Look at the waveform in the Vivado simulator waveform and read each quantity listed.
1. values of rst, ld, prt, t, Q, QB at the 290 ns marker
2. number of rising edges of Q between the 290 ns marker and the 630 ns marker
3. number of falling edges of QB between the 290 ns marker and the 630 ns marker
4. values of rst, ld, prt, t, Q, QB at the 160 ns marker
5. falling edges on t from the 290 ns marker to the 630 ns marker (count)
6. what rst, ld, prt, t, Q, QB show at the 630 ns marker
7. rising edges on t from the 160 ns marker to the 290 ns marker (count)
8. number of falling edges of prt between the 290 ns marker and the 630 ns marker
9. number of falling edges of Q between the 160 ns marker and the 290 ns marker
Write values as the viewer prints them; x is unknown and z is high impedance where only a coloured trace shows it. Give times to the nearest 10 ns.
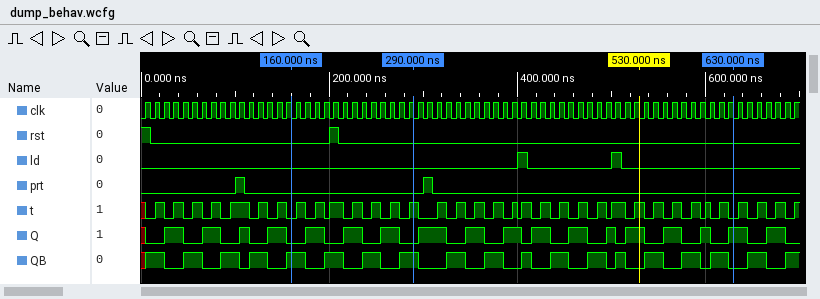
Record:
rst=0, ld=0, prt=0, t=1, Q=0, QB=1
10
10
rst=0, ld=0, prt=0, t=0, Q=0, QB=1
18
rst=0, ld=0, prt=0, t=0, Q=1, QB=0
7
1
3
